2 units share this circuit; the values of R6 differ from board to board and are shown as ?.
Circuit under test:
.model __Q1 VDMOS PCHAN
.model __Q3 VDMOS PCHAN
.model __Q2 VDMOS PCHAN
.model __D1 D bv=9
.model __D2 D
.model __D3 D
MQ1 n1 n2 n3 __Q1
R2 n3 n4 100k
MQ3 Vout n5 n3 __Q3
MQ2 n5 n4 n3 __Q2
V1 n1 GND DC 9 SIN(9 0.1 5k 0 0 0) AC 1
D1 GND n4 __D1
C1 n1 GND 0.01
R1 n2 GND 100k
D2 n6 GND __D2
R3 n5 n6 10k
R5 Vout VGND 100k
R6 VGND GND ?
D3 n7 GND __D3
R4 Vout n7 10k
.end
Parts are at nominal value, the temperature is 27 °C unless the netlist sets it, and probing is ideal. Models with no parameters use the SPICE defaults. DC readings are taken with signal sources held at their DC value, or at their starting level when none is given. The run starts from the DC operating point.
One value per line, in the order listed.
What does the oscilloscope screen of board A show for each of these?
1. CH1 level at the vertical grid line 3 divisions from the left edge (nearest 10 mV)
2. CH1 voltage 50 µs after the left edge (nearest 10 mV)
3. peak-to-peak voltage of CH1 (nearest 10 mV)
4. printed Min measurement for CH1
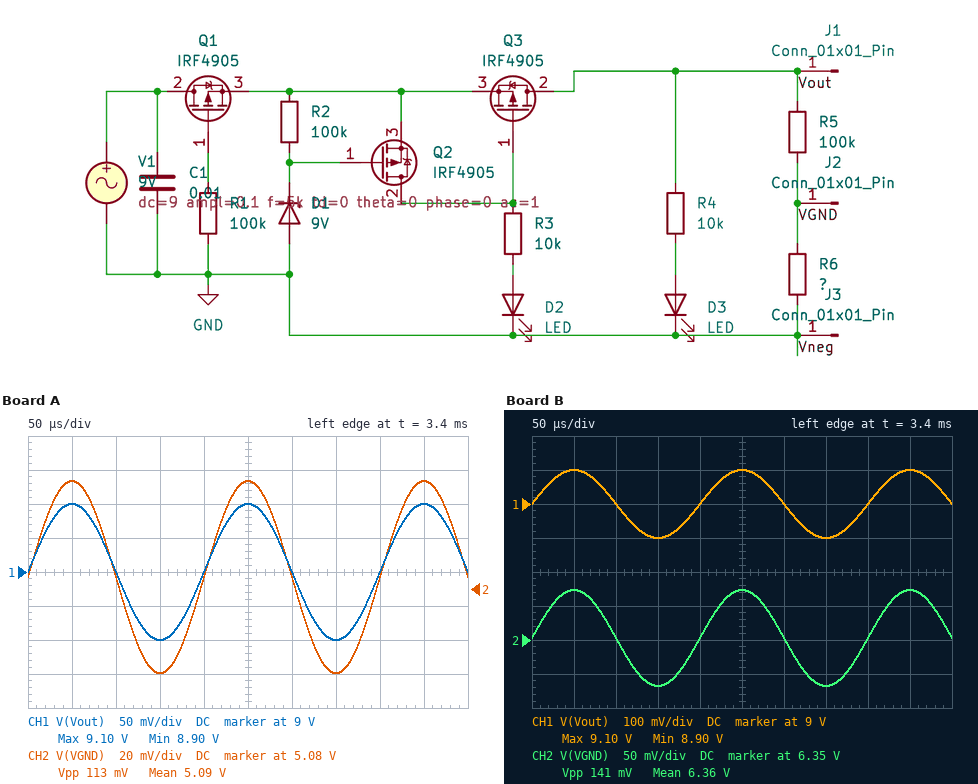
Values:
8.90 V
9.10 V
200 mV
8.90 V
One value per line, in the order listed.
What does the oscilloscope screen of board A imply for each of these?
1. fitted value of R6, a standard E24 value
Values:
130 kΩ
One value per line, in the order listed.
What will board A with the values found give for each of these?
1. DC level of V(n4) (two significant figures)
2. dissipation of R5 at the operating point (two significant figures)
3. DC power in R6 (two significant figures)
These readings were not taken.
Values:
8.8 V
150 µW
200 µW
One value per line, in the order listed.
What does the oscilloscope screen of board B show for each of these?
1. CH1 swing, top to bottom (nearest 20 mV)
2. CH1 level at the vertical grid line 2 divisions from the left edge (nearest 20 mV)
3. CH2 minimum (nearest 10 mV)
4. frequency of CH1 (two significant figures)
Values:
200 mV
9.00 V
6.28 V
5.0 kHz
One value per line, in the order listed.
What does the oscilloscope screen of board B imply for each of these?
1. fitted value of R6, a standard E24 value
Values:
240 kΩ
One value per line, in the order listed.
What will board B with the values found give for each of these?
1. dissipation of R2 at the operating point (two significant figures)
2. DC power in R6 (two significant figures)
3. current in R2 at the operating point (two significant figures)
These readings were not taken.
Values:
270 nW
170 µW
1.7 µA
